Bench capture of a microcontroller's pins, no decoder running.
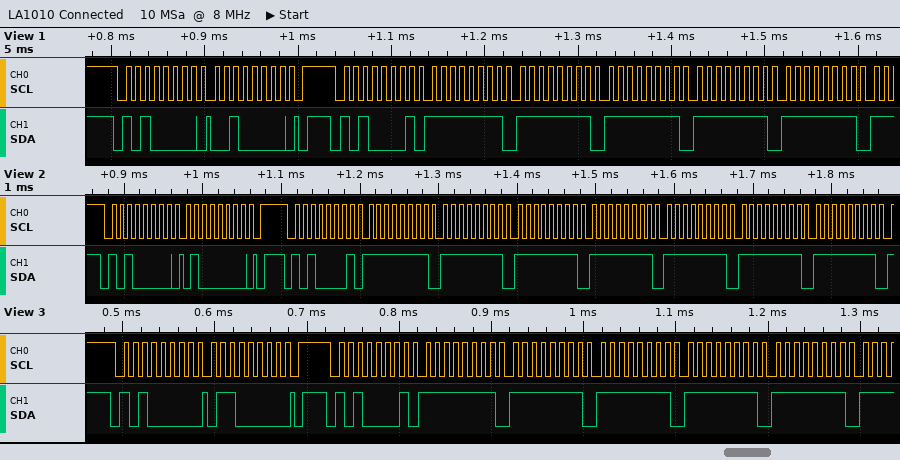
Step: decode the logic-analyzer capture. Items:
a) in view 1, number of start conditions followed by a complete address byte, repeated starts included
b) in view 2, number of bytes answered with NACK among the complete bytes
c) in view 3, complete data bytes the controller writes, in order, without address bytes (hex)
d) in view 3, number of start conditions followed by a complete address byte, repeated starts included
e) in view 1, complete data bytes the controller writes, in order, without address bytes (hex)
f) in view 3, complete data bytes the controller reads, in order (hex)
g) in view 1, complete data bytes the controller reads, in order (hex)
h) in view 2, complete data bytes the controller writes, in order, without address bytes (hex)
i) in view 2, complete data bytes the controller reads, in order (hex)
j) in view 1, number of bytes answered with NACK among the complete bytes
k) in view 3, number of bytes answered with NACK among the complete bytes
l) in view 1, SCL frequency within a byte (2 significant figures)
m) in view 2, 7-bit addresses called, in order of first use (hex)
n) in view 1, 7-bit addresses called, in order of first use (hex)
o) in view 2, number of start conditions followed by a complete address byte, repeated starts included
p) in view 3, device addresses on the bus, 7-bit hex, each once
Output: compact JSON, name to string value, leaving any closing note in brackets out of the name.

{"in view 1, number of start conditions followed by a complete address byte, repeated starts included": "2", "in view 2, number of bytes answered with NACK among the complete bytes": "0", "in view 3, complete data bytes the controller writes, in order, without address bytes": "60", "in view 3, number of start conditions followed by a complete address byte, repeated starts included": "2", "in view 1, complete data bytes the controller writes, in order, without address bytes": "20", "in view 3, complete data bytes the controller reads, in order": "FF FF FF FF FF", "in view 1, complete data bytes the controller reads, in order": "FF FF FF FF FF", "in view 2, complete data bytes the controller writes, in order, without address bytes": "40", "in view 2, complete data bytes the controller reads, in order": "FF FF FF FF FF FF FF", "in view 1, number of bytes answered with NACK among the complete bytes": "0", "in view 3, number of bytes answered with NACK among the complete bytes": "0", "in view 1, SCL frequency within a byte": "100 kHz", "in view 2, 7-bit addresses called, in order of first use": "0x50", "in view 1, 7-bit addresses called, in order of first use": "0x50", "in view 2, number of start conditions followed by a complete address byte, repeated starts included": "2", "in view 3, device addresses on the bus, 7-bit hex, each once": "0x50"}
